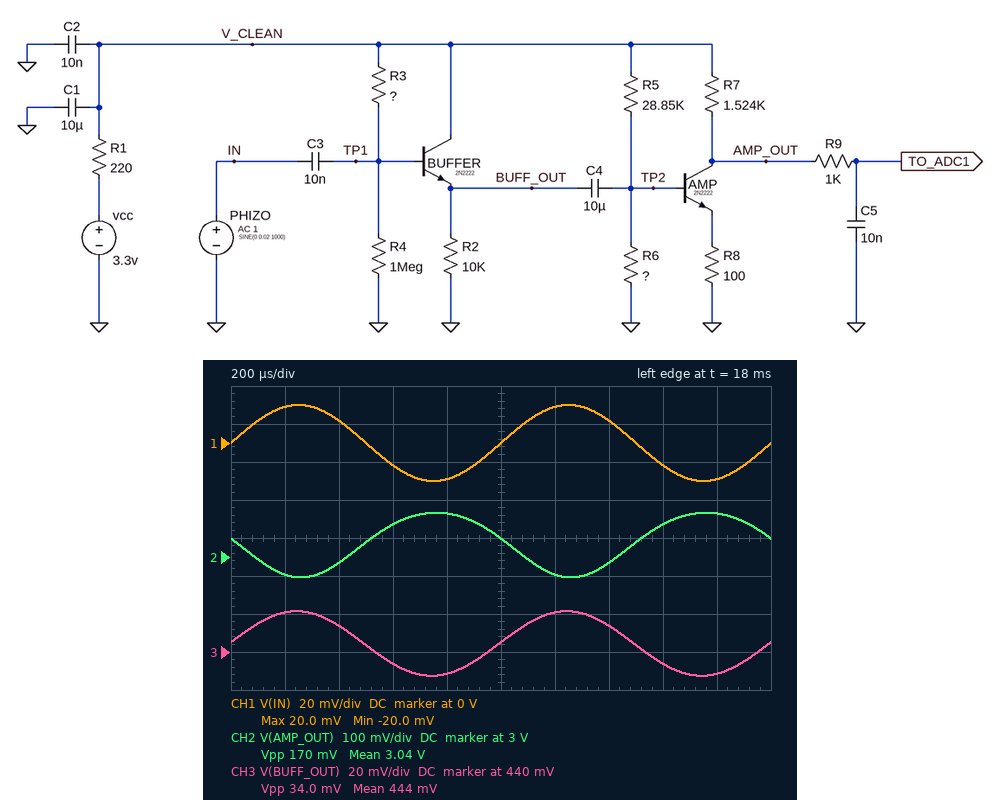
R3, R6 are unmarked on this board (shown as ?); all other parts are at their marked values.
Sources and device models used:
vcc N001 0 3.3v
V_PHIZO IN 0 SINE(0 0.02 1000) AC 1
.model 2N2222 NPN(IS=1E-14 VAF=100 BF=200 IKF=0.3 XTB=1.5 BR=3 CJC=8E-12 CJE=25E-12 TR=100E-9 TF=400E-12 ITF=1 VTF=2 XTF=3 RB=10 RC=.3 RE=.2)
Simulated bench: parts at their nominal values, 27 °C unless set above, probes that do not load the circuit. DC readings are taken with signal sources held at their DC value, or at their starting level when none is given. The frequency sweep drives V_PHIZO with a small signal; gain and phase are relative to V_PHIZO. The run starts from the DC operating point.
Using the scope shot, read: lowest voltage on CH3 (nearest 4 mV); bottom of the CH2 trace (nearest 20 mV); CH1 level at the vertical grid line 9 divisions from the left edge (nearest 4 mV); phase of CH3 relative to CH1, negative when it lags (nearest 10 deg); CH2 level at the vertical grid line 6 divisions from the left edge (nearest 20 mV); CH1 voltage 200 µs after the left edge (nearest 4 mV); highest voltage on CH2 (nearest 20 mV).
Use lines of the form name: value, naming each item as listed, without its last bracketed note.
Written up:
lowest voltage on CH3: 428 mV
bottom of the CH2 trace: 2.94 V
CH1 level at the vertical grid line 9 divisions from the left edge: -20 mV
phase of CH3 relative to CH1, negative when it lags: 0 deg
CH2 level at the vertical grid line 6 divisions from the left edge: 2.96 V
CH1 voltage 200 µs after the left edge: 20 mV
highest voltage on CH2: 3.12 V
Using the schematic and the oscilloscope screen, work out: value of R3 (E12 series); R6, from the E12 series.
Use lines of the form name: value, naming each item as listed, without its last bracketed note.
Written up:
value of R3: 1.8 MΩ
R6, from the E12 series: 6.8 kΩ
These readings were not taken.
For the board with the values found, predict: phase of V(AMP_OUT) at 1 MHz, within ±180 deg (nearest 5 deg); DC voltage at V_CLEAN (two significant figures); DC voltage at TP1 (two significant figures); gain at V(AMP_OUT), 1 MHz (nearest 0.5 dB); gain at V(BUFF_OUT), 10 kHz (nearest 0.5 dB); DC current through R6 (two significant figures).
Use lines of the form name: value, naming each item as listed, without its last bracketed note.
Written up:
phase of V(AMP_OUT) at 1 MHz, within ±180 deg: 170 deg
DC voltage at V_CLEAN: 3.2 V
DC voltage at TP1: 1.0 V
gain at V(AMP_OUT), 1 MHz: 4.5 dB
gain at V(BUFF_OUT), 10 kHz: -1.5 dB
DC current through R6: 90 µA
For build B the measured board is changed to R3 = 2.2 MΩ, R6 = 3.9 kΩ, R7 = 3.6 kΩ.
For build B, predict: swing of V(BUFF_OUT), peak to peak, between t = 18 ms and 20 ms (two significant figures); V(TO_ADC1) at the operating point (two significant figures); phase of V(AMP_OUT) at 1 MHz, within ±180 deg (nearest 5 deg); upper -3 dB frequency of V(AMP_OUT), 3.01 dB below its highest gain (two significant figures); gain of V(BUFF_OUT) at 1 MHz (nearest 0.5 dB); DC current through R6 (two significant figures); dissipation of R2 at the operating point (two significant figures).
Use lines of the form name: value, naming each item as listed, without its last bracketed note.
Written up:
swing of V(BUFF_OUT), peak to peak, between t = 18 ms and 20 ms: 31 mV
V(TO_ADC1) at the operating point: 3.3 V
phase of V(AMP_OUT) at 1 MHz, within ±180 deg: 85 deg
upper -3 dB frequency of V(AMP_OUT), 3.01 dB below its highest gain: 3.6 GHz
gain of V(BUFF_OUT) at 1 MHz: -2.5 dB
DC current through R6: 100 µA
dissipation of R2 at the operating point: 12 µW
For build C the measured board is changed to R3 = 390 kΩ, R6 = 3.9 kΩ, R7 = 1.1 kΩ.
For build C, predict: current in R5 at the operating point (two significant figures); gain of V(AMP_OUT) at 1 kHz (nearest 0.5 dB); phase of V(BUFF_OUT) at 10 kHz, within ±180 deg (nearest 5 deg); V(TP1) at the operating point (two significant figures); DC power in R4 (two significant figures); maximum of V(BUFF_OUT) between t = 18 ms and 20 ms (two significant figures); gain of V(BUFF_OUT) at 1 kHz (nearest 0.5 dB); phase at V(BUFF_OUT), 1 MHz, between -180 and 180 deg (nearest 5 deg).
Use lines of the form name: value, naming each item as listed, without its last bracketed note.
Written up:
current in R5 at the operating point: 99 µA
gain of V(AMP_OUT) at 1 kHz: -45.5 dB
phase of V(BUFF_OUT) at 10 kHz, within ±180 deg: 0 deg
V(TP1) at the operating point: 2.1 V
DC power in R4: 4.5 µW
maximum of V(BUFF_OUT) between t = 18 ms and 20 ms: 1.5 V
gain of V(BUFF_OUT) at 1 kHz: -0.5 dB
phase at V(BUFF_OUT), 1 MHz, between -180 and 180 deg: 0 deg
